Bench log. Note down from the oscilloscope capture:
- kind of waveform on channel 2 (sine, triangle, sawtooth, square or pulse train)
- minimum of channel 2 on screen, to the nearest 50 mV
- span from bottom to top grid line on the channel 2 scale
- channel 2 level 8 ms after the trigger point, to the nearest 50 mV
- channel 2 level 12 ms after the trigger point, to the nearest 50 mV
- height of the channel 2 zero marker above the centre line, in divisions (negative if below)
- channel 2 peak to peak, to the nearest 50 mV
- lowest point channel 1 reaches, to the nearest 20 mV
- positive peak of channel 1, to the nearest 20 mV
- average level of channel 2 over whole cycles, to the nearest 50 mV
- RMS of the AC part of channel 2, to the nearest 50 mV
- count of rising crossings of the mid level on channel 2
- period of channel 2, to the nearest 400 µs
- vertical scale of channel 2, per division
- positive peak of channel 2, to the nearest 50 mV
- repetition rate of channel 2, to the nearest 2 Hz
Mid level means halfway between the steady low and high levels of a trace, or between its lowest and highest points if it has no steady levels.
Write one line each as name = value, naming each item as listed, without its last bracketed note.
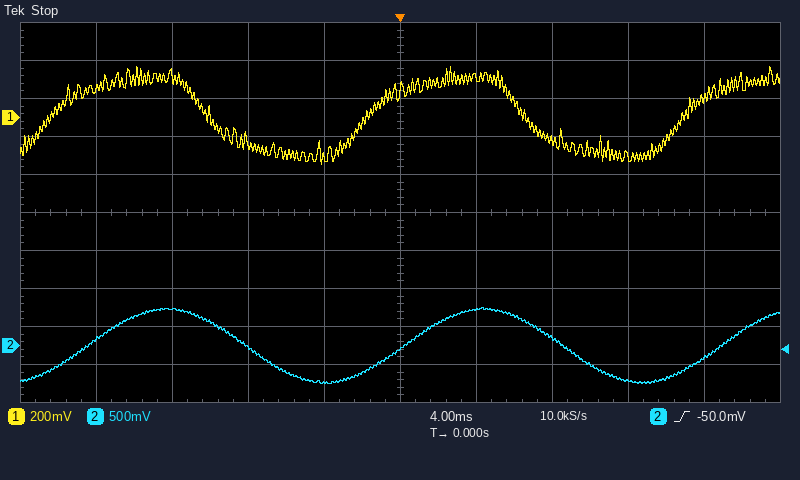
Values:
kind of waveform on channel 2 = sine
minimum of channel 2 on screen, to the nearest 50 mV = -500 mV
span from bottom to top grid line on the channel 2 scale = 5 V
channel 2 level 8 ms after the trigger point, to the nearest 50 mV = 100 mV
channel 2 level 12 ms after the trigger point, to the nearest 50 mV = -450 mV
height of the channel 2 zero marker above the centre line, in divisions = -3.5 div
channel 2 peak to peak, to the nearest 50 mV = 1.00 V
lowest point channel 1 reaches, to the nearest 20 mV = -240 mV
positive peak of channel 1, to the nearest 20 mV = 260 mV
average level of channel 2 over whole cycles, to the nearest 50 mV = 0 mV
RMS of the AC part of channel 2, to the nearest 50 mV = 350 mV
count of rising crossings of the mid level on channel 2 = 3
period of channel 2, to the nearest 400 µs = 16.8 ms
vertical scale of channel 2, per division = 500 mV
positive peak of channel 2, to the nearest 50 mV = 500 mV
repetition rate of channel 2, to the nearest 2 Hz = 60 Hz
